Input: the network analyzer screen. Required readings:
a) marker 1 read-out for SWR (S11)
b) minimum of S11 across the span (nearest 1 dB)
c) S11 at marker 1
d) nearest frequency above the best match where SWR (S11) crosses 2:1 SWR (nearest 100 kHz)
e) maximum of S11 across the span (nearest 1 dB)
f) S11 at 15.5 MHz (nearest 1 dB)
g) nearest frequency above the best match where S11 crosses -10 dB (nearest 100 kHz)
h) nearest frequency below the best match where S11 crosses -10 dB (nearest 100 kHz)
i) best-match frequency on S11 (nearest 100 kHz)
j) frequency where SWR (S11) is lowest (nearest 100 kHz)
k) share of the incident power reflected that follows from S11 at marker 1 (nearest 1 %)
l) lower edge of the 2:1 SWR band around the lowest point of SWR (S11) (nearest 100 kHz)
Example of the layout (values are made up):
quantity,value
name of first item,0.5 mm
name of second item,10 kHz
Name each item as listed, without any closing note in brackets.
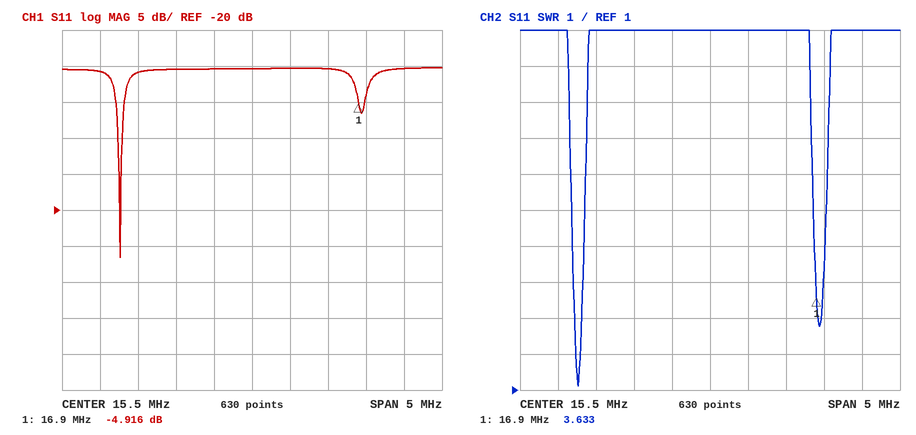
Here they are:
quantity,value
marker 1 read-out for SWR,3.633
minimum of S11 across the span,-27 dB
S11 at marker 1,-4.916 dB
nearest frequency above the best match where SWR (S11) crosses 2:1 SWR,13.8 MHz
maximum of S11 across the span,0 dB
S11 at 15.5 MHz,0 dB
nearest frequency above the best match where S11 crosses -10 dB,13.8 MHz
nearest frequency below the best match where S11 crosses -10 dB,13.7 MHz
best-match frequency on S11,13.8 MHz
frequency where SWR (S11) is lowest,13.8 MHz
share of the incident power reflected that follows from S11 at marker 1,32 %
lower edge of the 2:1 SWR band around the lowest point of SWR (S11),13.7 MHz
